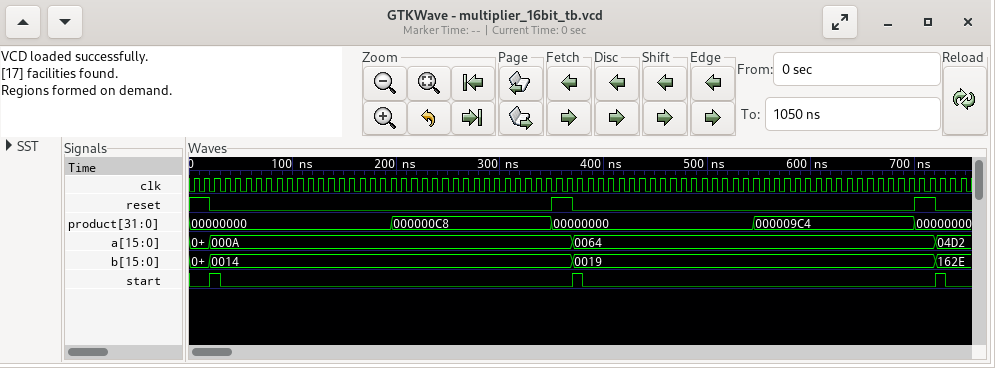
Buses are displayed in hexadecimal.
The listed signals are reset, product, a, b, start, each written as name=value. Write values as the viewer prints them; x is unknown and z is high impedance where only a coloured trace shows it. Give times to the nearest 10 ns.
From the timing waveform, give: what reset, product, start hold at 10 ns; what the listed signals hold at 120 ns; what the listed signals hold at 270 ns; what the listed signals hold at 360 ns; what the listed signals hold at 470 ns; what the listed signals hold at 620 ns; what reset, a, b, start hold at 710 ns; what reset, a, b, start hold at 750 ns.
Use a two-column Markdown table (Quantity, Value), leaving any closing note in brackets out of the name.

| Quantity | Value |
|---|---|
| what reset, product, start hold at 10 ns | reset=1, product=00000000, start=0 |
| what the listed signals hold at 120 ns | reset=0, product=00000000, a=000A, b=0014, start=0 |
| what the listed signals hold at 270 ns | reset=0, product=000000C8, a=000A, b=0014, start=0 |
| what the listed signals hold at 360 ns | reset=1, product=00000000, a=000A, b=0014, start=0 |
| what the listed signals hold at 470 ns | reset=0, product=00000000, a=0064, b=0019, start=0 |
| what the listed signals hold at 620 ns | reset=0, product=000009C4, a=0064, b=0019, start=0 |
| what reset, a, b, start hold at 710 ns | reset=1, a=0064, b=0019, start=0 |
| what reset, a, b, start hold at 750 ns | reset=0, a=04D2, b=162E, start=0 |
